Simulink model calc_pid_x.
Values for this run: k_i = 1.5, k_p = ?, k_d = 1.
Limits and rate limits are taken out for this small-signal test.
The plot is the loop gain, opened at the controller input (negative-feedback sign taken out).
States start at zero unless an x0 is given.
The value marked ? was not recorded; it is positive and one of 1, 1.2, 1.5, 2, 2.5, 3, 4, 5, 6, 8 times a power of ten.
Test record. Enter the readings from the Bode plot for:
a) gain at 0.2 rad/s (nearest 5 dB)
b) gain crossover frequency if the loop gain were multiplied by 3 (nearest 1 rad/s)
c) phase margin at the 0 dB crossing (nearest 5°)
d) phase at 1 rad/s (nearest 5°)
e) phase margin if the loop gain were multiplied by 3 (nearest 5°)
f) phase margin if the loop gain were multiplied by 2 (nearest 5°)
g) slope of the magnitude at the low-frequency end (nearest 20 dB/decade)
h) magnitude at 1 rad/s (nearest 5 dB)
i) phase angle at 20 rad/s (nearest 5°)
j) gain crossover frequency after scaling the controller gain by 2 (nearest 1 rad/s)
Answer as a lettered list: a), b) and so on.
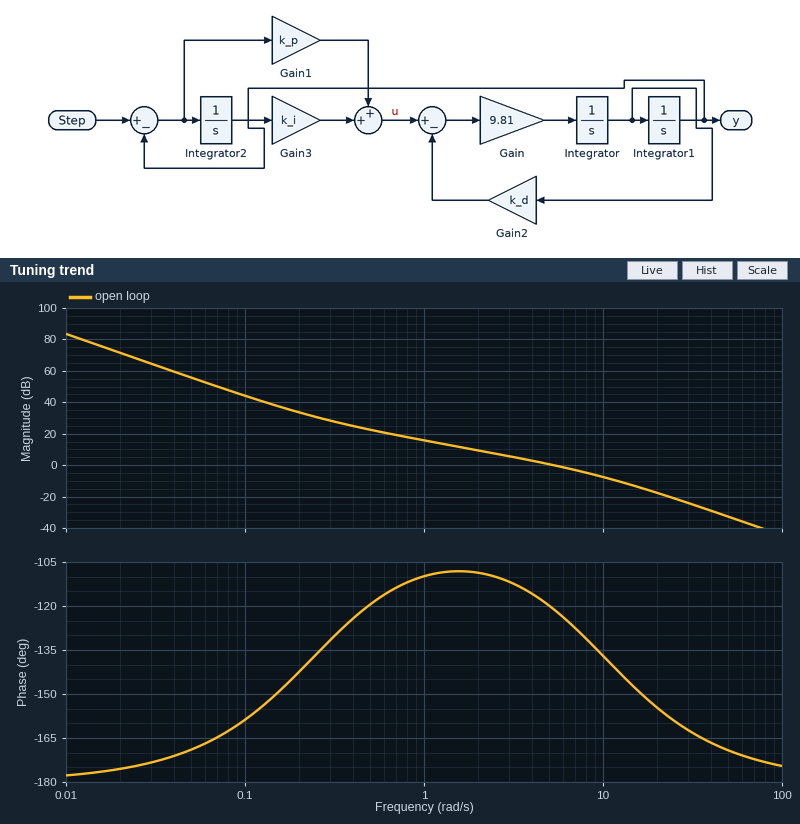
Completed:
a) 35 dB
b) 12 rad/s
c) 60°
d) -110°
e) 40°
f) 45°
g) -40 dB/decade
h) 15 dB
i) -155°
j) 9 rad/s
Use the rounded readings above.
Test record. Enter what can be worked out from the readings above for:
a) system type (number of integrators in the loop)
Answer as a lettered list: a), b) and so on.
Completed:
a) 2
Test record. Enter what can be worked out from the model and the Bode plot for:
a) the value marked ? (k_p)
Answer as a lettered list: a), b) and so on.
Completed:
a) 6
